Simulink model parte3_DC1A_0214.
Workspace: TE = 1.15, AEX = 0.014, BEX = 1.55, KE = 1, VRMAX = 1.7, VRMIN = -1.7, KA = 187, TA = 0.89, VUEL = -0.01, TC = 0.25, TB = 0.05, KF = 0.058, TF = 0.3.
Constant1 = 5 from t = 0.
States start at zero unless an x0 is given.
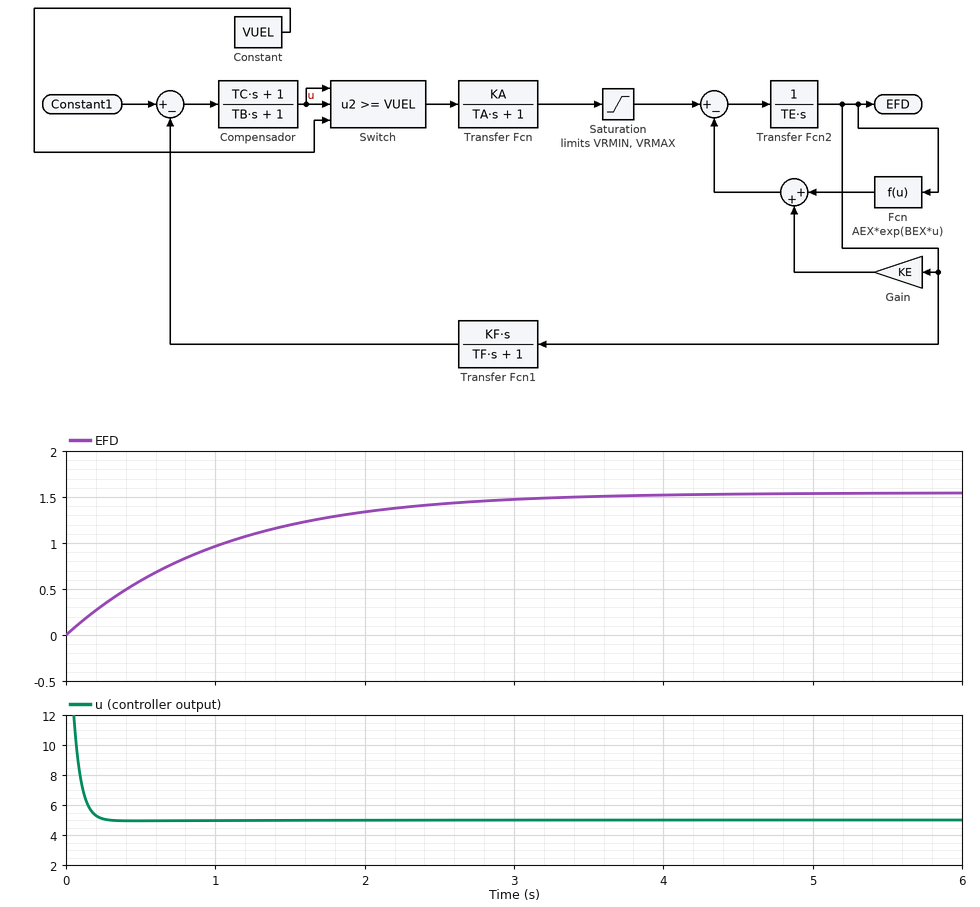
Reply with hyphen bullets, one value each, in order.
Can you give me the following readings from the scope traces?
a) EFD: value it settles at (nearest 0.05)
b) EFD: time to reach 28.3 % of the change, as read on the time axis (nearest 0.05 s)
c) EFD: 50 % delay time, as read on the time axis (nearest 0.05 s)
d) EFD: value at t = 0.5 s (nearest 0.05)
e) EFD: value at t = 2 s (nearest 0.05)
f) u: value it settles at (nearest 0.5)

- 1.55
- 0.35 s
- 0.70 s
- 0.60
- 1.35
- 5.0
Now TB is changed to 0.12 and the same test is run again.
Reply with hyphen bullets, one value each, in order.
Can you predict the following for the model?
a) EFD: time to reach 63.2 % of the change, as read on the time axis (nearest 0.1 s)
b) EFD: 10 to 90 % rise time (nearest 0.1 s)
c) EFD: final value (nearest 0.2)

- 1.0 s
- 2.2 s
- 1.6
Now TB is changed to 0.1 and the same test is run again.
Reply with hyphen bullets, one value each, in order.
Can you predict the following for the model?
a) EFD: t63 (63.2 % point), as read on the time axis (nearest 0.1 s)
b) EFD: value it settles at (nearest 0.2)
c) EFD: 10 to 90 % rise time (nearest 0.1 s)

- 1.0 s
- 1.6
- 2.2 s
